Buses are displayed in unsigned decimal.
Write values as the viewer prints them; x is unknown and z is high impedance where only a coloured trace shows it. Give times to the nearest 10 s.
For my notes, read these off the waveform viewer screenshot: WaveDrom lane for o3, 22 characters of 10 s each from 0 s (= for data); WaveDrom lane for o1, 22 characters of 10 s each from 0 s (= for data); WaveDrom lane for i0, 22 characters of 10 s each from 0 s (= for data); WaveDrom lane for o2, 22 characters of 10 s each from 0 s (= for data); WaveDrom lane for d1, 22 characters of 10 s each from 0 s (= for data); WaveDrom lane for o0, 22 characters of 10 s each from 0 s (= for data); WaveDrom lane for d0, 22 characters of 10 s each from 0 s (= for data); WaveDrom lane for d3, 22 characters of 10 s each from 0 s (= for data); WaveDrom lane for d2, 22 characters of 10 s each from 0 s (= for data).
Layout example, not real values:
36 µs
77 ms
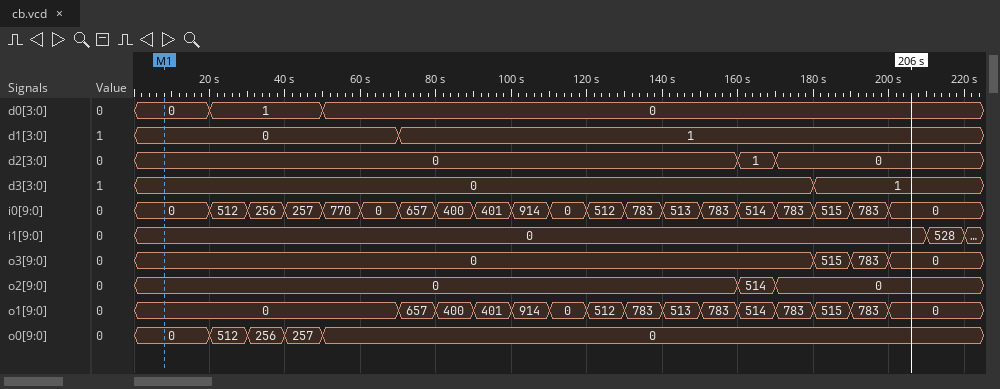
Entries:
{name: 'o3', wave: '=.................===.', data: '0 515 783 0'}
{name: 'o1', wave: '=......==============.', data: '0 657 400 401 914 0 512 783 513 783 514 783 515 783 0'}
{name: 'i0', wave: '=.===================.', data: '0 512 256 257 770 0 657 400 401 914 0 512 783 513 783 514 783 515 783 0'}
{name: 'o2', wave: '=...............==....', data: '0 514 0'}
{name: 'd1', wave: '=......=..............', data: '0 1'}
{name: 'o0', wave: '=.====................', data: '0 512 256 257 0'}
{name: 'd0', wave: '=.=..=................', data: '0 1 0'}
{name: 'd3', wave: '=.................=...', data: '0 1'}
{name: 'd2', wave: '=...............==....', data: '0 1 0'}
